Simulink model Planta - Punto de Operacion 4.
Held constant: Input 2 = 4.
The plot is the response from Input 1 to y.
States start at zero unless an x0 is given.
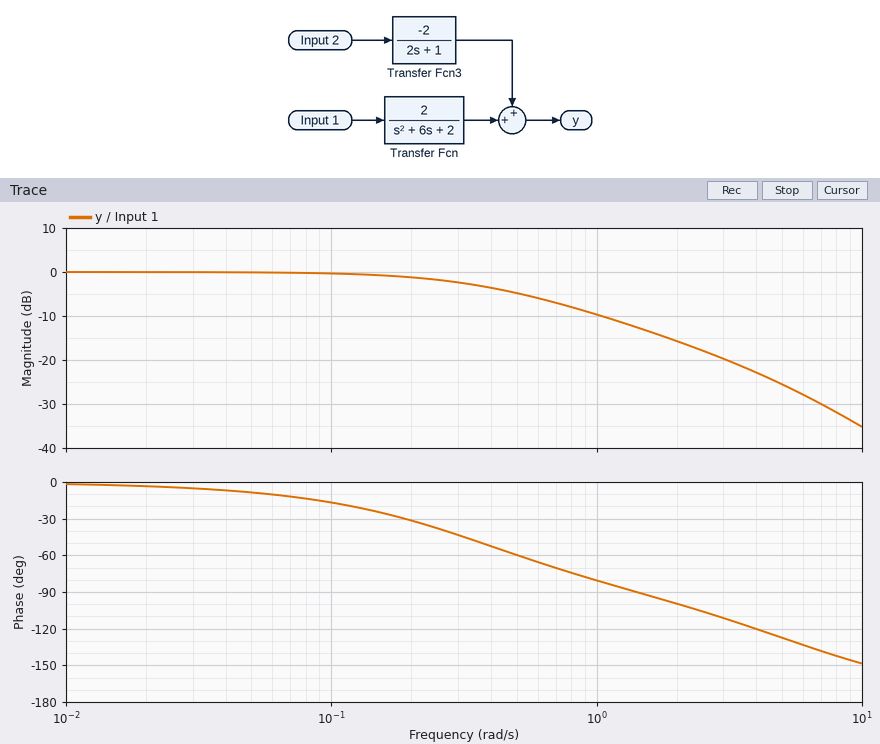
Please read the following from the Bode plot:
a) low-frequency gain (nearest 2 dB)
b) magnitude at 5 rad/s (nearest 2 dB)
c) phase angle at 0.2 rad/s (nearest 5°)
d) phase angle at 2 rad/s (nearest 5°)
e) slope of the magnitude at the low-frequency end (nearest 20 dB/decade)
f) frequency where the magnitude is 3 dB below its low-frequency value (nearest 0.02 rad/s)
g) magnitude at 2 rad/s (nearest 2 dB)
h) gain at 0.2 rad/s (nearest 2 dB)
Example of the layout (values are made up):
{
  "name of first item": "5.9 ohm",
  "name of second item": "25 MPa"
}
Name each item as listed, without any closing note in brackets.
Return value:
{
  "low-frequency gain": "0 dB",
  "magnitude at 5 rad/s": "-26 dB",
  "phase angle at 0.2 rad/s": "-30°",
  "phase angle at 2 rad/s": "-100°",
  "slope of the magnitude at the low-frequency end": "0 dB/decade",
  "frequency where the magnitude is 3 dB below its low-frequency value": "0.36 rad/s",
  "magnitude at 2 rad/s": "-16 dB",
  "gain at 0.2 rad/s": "-2 dB"
}
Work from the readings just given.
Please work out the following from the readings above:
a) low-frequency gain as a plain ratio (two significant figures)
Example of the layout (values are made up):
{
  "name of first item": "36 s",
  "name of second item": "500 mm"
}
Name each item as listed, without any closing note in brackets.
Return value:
{
  "low-frequency gain as a plain ratio": "1.0"
}
